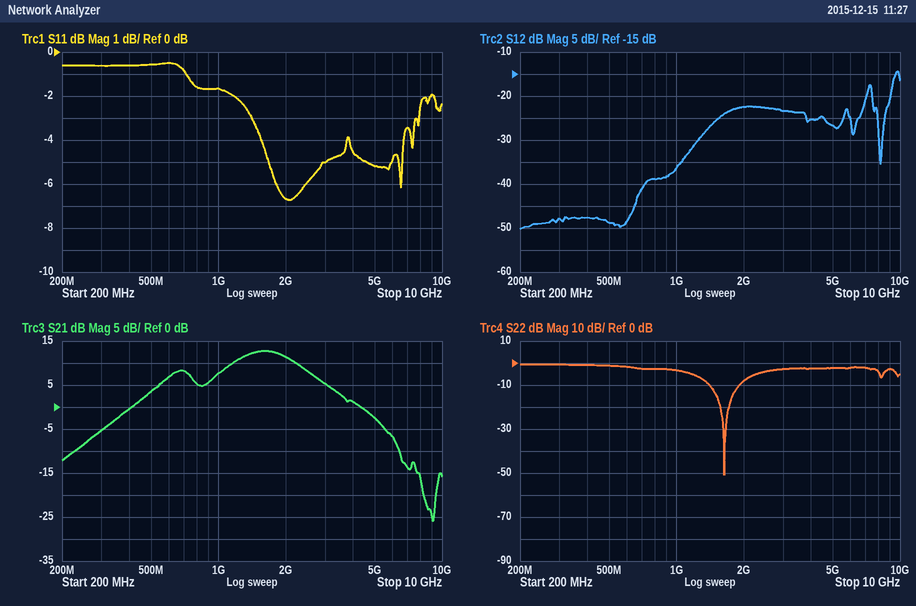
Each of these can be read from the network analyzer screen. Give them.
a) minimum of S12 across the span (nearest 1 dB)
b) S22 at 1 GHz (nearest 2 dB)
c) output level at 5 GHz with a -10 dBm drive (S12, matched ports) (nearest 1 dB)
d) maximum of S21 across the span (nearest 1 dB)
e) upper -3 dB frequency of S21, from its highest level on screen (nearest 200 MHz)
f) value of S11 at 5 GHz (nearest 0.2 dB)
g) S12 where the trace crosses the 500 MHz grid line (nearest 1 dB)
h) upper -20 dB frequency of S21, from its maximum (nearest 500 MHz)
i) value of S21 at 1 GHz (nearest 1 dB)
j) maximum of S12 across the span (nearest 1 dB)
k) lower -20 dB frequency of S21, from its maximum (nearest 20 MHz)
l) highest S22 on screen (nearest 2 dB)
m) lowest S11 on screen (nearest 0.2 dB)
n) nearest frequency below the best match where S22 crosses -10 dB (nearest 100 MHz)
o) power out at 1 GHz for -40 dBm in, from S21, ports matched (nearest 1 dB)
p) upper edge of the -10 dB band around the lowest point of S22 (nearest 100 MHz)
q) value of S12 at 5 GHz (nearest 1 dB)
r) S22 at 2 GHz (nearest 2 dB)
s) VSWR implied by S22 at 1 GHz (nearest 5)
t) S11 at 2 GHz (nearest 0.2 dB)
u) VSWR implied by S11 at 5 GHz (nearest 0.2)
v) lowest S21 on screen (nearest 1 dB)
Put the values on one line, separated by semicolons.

-50 dB; -4 dB; -37 dBm; 13 dB; 2.2 GHz; -5.2 dB; -49 dB; 6.0 GHz; 8 dB; -14 dB; 260 MHz; 0 dB; -6.8 dB; 1.4 GHz; -32 dBm; 1.9 GHz; -27 dB; -8 dB; 5; -6.6 dB; 3.4; -26 dB
